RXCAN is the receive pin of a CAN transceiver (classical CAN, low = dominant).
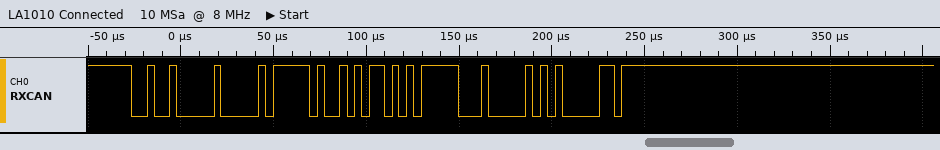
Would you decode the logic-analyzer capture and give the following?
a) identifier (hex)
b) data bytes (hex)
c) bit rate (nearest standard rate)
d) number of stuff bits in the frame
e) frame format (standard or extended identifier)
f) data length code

0x240
F2 B5 7C
250 kbit/s
6
standard
3
